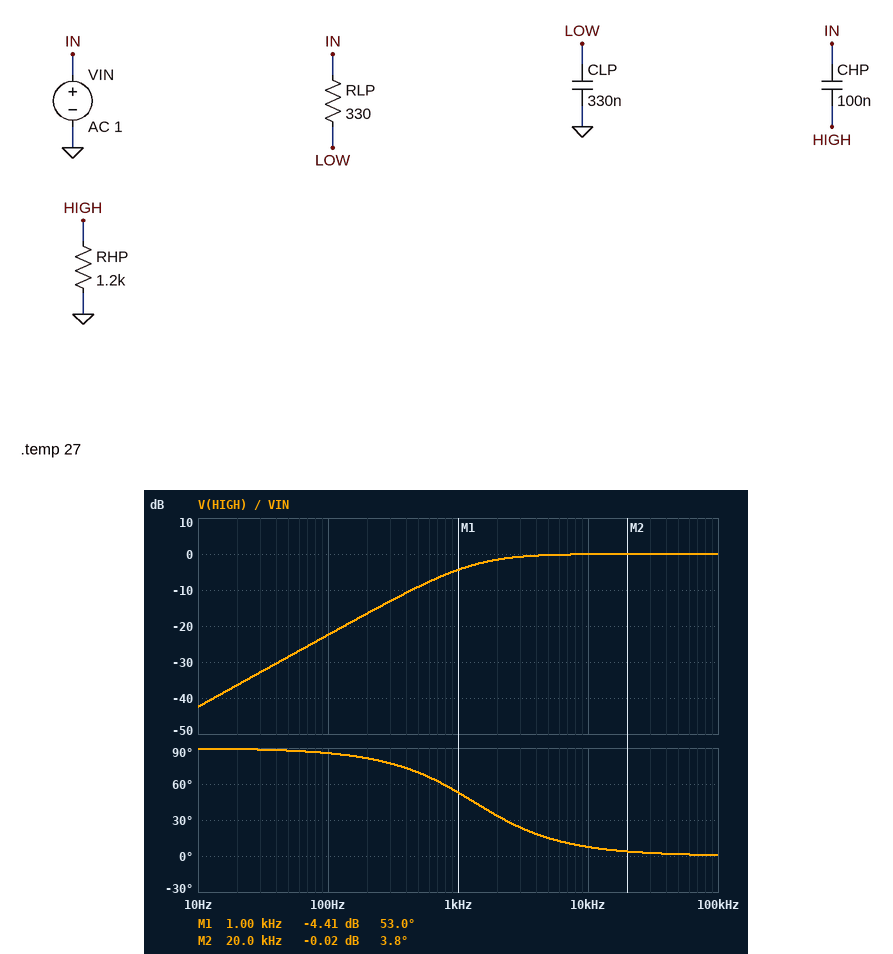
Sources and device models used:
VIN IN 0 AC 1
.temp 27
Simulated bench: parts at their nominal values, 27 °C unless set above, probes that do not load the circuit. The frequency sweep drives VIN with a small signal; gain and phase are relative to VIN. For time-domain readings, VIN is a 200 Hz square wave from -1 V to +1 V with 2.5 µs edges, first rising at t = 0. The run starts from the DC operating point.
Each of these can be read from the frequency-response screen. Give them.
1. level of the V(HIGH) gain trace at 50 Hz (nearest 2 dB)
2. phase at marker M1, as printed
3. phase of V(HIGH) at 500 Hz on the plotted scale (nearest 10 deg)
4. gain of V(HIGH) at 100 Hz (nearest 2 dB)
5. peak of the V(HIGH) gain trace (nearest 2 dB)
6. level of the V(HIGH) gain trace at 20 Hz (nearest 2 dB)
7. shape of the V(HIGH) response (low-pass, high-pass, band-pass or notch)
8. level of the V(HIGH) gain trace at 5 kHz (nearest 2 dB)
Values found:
-28 dB
53.0 deg
70 deg
-22 dB
0 dB
-36 dB
high-pass
0 dB
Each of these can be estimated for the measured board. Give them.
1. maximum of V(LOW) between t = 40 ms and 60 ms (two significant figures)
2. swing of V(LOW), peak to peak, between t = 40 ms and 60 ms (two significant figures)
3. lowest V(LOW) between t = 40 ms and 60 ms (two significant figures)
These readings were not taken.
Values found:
1.0 V
2.0 V
-1.0 V
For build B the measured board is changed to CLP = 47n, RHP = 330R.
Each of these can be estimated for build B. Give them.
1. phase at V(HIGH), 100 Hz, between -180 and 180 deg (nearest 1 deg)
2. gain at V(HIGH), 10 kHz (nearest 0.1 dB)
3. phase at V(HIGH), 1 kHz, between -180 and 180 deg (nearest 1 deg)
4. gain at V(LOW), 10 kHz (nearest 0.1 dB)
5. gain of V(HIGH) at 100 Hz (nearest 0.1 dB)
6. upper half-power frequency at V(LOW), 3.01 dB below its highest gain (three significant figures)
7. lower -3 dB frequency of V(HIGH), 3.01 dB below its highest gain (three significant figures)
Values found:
89 deg
-0.9 dB
78 deg
-2.9 dB
-33.7 dB
10.3 kHz
4.82 kHz
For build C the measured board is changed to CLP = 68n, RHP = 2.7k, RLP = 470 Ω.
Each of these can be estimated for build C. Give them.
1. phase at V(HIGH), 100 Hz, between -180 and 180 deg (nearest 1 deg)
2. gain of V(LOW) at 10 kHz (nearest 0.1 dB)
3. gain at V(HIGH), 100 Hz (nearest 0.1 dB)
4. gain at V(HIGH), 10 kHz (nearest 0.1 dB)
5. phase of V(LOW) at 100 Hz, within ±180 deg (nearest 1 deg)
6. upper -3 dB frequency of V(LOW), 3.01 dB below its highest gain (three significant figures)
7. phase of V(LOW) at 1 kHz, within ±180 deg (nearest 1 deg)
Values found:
80 deg
-7.0 dB
-15.5 dB
0 dB
-1 deg
4.98 kHz
-11 deg
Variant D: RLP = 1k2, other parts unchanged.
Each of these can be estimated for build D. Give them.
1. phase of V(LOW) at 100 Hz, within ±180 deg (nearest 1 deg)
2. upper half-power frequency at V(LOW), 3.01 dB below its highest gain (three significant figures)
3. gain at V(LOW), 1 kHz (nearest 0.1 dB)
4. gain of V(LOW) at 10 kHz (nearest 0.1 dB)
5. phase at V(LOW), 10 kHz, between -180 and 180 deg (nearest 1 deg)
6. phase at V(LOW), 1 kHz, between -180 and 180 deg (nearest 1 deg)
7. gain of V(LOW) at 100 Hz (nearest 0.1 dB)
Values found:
-14 deg
402 Hz
-8.6 dB
-27.9 dB
-88 deg
-68 deg
-0.3 dB
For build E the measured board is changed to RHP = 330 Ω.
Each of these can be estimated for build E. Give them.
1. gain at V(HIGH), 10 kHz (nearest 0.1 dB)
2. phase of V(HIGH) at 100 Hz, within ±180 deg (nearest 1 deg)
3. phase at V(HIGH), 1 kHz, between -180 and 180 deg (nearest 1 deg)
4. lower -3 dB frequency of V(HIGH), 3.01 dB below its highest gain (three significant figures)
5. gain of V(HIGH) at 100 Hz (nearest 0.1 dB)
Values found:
-0.9 dB
89 deg
78 deg
4.82 kHz
-33.7 dB
